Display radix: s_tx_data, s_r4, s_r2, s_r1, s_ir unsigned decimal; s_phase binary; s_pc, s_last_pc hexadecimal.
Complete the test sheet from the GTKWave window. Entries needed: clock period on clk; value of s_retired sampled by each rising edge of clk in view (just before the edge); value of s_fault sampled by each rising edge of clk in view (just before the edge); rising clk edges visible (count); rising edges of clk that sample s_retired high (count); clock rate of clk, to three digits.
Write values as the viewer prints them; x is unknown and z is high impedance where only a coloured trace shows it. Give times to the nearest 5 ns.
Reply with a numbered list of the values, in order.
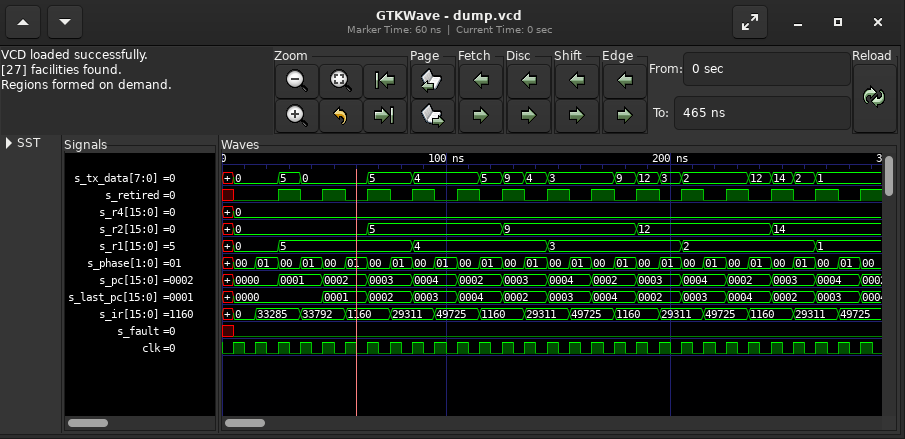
1. 10 ns
2. x 0 0 1 0 1 0 1 0 1 0 1 0 1 0 1 0 1 0 1 0 1 0 1 0 1 0 1 0
3. x 0 0 0 0 0 0 0 0 0 0 0 0 0 0 0 0 0 0 0 0 0 0 0 0 0 0 0 0
4. 29
5. 13
6. 100 MHz
